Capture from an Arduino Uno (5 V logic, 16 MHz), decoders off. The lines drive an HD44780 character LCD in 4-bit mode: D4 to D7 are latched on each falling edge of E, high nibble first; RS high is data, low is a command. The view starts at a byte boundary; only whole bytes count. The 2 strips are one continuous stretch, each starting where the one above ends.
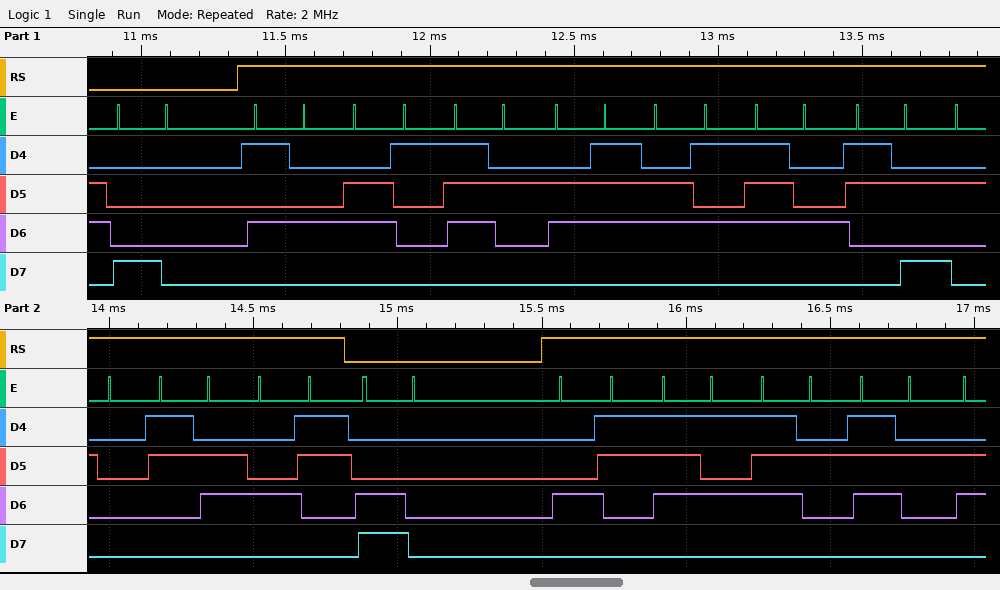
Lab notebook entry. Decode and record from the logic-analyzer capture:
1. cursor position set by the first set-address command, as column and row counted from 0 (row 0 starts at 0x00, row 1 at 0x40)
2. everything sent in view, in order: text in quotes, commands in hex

column 0, row 0
0x80 "Target: 6C" 0xC0 "Curr"
